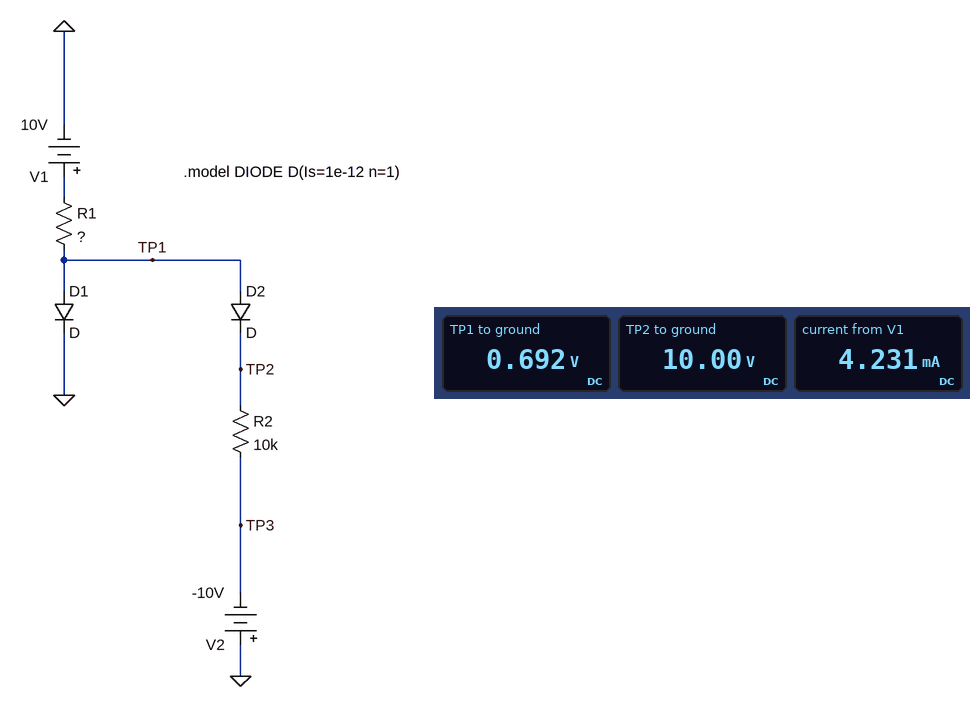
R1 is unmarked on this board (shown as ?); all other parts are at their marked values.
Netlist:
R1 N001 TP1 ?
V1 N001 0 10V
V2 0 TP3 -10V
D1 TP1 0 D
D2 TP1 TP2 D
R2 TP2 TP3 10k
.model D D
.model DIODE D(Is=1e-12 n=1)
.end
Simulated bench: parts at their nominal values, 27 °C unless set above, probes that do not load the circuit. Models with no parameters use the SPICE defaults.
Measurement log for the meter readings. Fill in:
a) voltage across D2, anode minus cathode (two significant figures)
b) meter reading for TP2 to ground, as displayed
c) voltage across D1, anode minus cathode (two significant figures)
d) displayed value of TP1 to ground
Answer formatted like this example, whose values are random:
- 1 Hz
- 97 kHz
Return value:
- -9.3 V
- 10.00 V
- 690 mV
- 0.692 V
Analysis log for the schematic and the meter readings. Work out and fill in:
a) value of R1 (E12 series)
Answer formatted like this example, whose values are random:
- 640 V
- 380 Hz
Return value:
- 2.2 kΩ
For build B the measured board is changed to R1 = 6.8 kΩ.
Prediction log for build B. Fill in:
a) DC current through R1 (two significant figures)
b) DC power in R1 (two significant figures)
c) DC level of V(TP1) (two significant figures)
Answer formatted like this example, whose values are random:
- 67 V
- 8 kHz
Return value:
- 1.4 mA
- 13 mW
- 660 mV
